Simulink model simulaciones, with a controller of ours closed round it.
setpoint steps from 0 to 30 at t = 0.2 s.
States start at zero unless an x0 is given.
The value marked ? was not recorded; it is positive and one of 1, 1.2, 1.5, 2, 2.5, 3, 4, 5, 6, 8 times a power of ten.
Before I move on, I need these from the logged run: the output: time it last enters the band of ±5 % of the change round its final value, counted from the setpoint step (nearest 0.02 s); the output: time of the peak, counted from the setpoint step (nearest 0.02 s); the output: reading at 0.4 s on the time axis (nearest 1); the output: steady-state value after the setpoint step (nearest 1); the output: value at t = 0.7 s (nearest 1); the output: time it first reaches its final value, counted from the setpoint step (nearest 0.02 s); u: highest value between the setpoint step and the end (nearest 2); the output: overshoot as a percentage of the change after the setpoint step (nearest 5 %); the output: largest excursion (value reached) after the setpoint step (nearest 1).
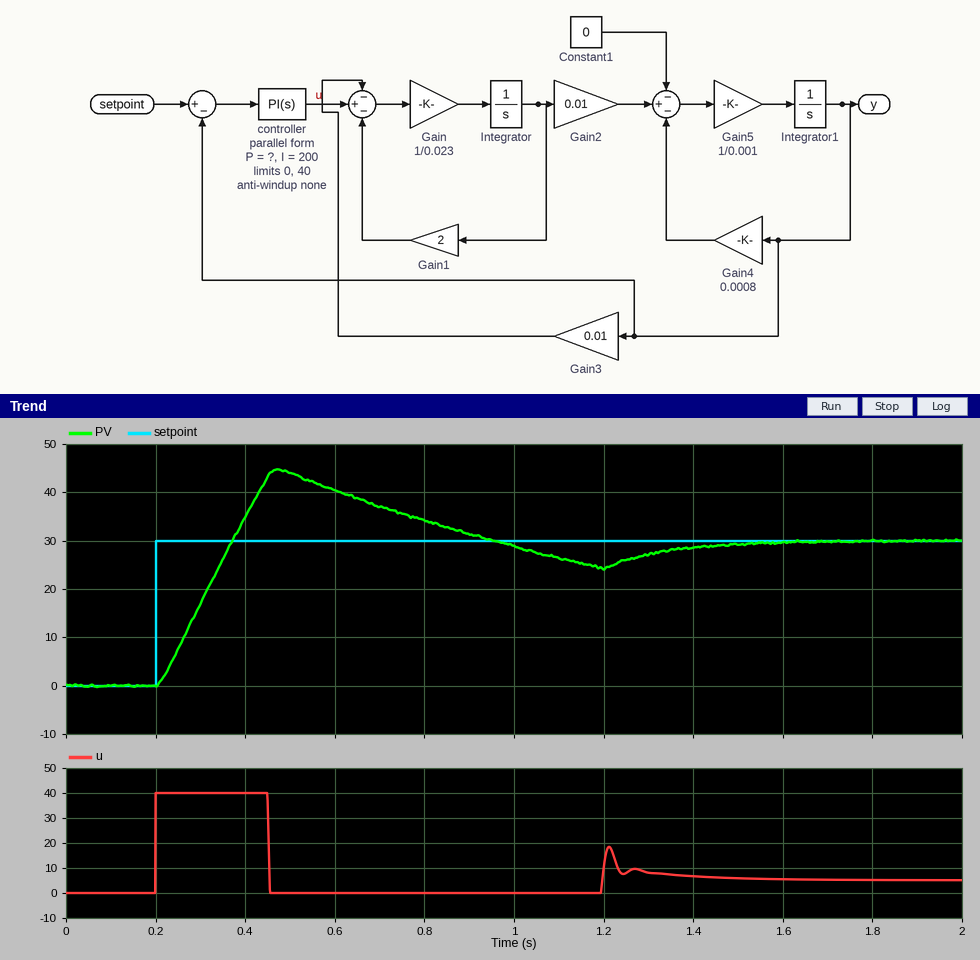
1.20 s
0.28 s
35
30
37
0.18 s
40
50 %
45
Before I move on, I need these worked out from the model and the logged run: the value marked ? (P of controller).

30
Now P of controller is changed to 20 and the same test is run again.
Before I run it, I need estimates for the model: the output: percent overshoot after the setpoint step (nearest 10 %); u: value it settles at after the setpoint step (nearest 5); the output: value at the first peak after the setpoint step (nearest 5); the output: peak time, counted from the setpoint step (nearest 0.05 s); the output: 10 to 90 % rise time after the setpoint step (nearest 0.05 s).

60 %
5
50
0.30 s
0.15 s
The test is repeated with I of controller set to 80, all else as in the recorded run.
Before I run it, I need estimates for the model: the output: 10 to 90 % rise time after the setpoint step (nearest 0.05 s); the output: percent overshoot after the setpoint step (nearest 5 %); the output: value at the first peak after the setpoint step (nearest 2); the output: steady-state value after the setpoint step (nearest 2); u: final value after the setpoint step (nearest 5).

0.15 s
25 %
38
30
5
